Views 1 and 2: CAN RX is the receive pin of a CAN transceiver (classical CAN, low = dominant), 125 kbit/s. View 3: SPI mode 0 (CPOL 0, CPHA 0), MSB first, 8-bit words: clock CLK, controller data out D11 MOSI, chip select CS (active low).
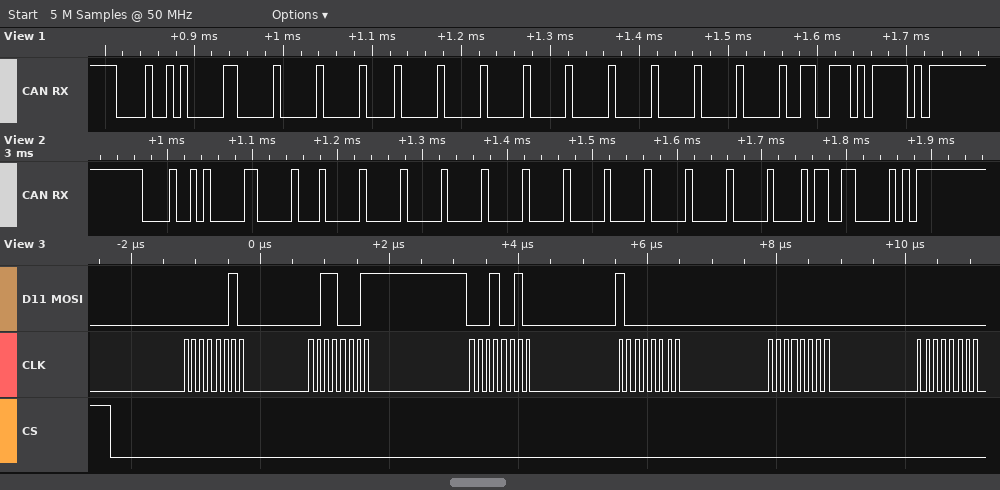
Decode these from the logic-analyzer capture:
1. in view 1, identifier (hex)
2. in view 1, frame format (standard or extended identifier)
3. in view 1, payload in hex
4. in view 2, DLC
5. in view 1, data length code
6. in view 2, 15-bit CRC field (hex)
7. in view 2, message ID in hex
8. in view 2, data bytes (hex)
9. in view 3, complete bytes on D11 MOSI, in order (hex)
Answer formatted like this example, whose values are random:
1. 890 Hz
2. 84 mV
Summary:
1. 0x094
2. standard
3. 00 00 80 00 00 00 00 00
4. 8
5. 8
6. 0x2CC0
7. 0x094
8. 04 00 00 00 00 00 00 00
9. 02 31 12 80 00 00
